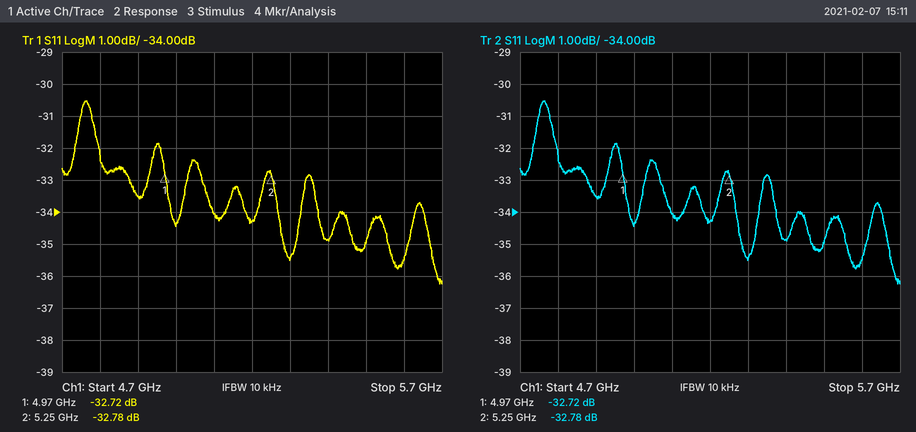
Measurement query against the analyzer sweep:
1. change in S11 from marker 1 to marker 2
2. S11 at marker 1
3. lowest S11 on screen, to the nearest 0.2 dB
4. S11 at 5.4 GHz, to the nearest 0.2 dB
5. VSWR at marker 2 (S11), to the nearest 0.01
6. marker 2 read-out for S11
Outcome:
-0.06 dB
-32.72 dB
-36.2 dB
-34.8 dB
1.05
-32.78 dB
